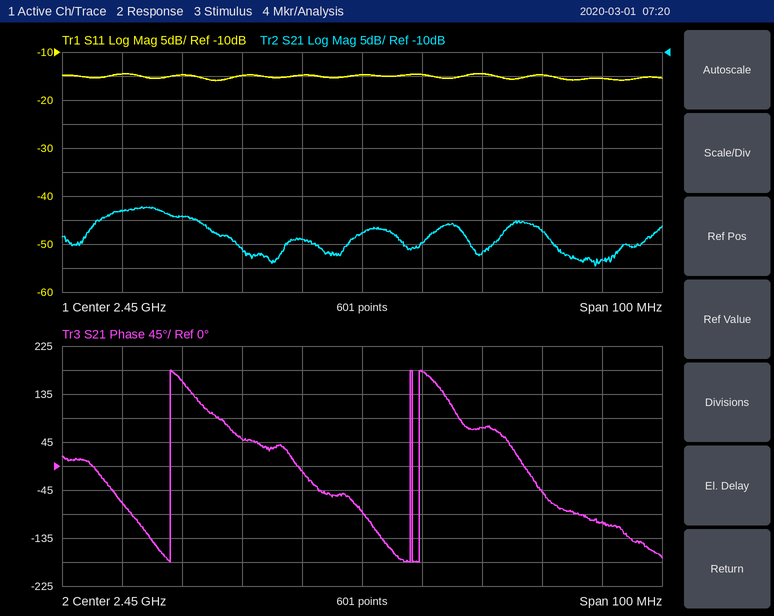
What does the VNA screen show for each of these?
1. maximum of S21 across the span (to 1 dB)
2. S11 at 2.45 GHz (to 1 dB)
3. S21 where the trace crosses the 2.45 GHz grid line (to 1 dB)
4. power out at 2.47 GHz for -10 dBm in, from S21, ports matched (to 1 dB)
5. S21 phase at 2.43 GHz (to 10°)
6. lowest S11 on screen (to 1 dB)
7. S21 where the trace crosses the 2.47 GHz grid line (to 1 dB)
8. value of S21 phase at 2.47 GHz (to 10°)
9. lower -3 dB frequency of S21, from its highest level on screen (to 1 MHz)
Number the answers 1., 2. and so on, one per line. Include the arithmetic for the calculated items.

1. -42 dB
2. -15 dB
3. -48 dB
4. -10 dBm + (-52 dB) = -62 dBm
5. 50°
6. -16 dB
7. -52 dB
8. 70°
9. 2.406 GHz
